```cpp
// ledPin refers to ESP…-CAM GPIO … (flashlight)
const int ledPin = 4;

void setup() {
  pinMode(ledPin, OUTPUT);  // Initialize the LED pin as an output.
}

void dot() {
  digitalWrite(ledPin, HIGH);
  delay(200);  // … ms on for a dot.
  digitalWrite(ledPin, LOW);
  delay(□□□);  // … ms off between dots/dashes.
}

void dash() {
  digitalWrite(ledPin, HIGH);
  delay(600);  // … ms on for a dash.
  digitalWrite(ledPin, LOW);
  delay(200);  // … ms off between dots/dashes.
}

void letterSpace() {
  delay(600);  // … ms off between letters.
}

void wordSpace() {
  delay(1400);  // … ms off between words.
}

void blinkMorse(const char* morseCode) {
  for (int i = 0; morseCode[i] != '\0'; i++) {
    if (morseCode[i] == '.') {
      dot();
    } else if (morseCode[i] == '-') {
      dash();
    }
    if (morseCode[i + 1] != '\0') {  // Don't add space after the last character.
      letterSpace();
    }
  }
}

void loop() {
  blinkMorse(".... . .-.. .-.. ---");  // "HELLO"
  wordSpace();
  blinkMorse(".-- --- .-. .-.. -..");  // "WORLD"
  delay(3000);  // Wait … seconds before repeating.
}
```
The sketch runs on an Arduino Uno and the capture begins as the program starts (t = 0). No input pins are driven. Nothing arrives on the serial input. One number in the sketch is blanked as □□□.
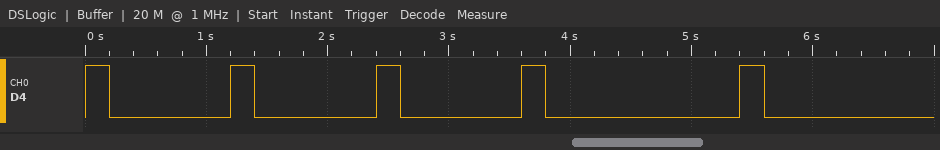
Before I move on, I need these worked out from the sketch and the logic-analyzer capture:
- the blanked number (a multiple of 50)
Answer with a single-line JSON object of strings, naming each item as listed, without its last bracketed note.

{"the blanked number": "400"}
